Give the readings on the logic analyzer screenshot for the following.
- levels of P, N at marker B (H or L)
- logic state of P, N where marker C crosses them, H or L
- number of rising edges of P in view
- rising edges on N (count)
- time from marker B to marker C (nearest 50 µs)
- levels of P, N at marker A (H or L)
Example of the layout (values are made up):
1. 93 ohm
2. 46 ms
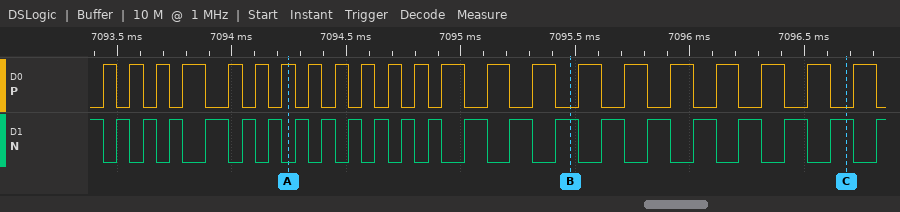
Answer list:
1. P=L, N=H
2. P=L, N=H
3. 22
4. 22
5. 1200 µs
6. P=H, N=L
